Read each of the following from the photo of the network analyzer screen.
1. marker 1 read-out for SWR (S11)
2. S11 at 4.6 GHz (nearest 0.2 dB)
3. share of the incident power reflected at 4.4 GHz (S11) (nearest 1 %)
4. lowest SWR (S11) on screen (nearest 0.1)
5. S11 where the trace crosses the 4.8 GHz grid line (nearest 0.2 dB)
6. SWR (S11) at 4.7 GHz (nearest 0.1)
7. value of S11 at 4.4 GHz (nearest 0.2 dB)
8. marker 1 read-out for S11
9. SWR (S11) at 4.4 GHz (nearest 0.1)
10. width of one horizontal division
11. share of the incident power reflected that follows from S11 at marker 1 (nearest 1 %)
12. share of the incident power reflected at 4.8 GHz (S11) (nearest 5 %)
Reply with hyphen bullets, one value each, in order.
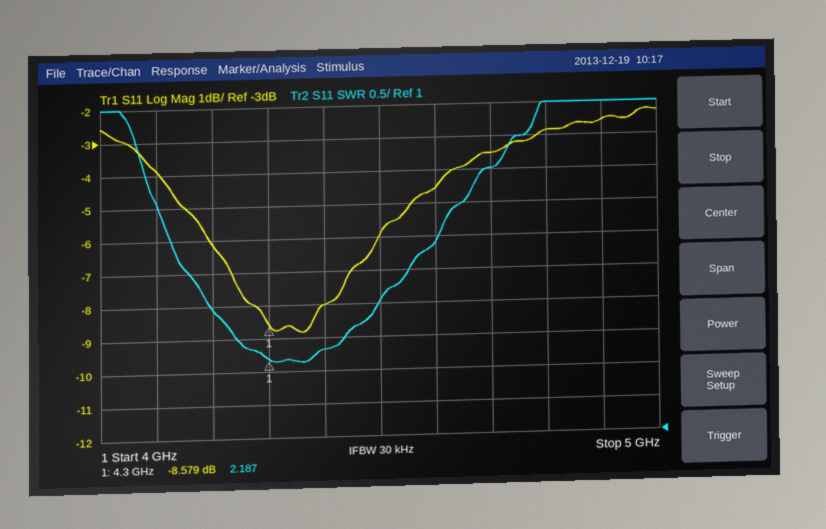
- 2.187
- -4.6 dB
- 16 %
- 2.1
- -2.8 dB
- 5.0
- -8.0 dB
- -8.579 dB
- 2.3
- 100 MHz
- 14 %
- 50 %
